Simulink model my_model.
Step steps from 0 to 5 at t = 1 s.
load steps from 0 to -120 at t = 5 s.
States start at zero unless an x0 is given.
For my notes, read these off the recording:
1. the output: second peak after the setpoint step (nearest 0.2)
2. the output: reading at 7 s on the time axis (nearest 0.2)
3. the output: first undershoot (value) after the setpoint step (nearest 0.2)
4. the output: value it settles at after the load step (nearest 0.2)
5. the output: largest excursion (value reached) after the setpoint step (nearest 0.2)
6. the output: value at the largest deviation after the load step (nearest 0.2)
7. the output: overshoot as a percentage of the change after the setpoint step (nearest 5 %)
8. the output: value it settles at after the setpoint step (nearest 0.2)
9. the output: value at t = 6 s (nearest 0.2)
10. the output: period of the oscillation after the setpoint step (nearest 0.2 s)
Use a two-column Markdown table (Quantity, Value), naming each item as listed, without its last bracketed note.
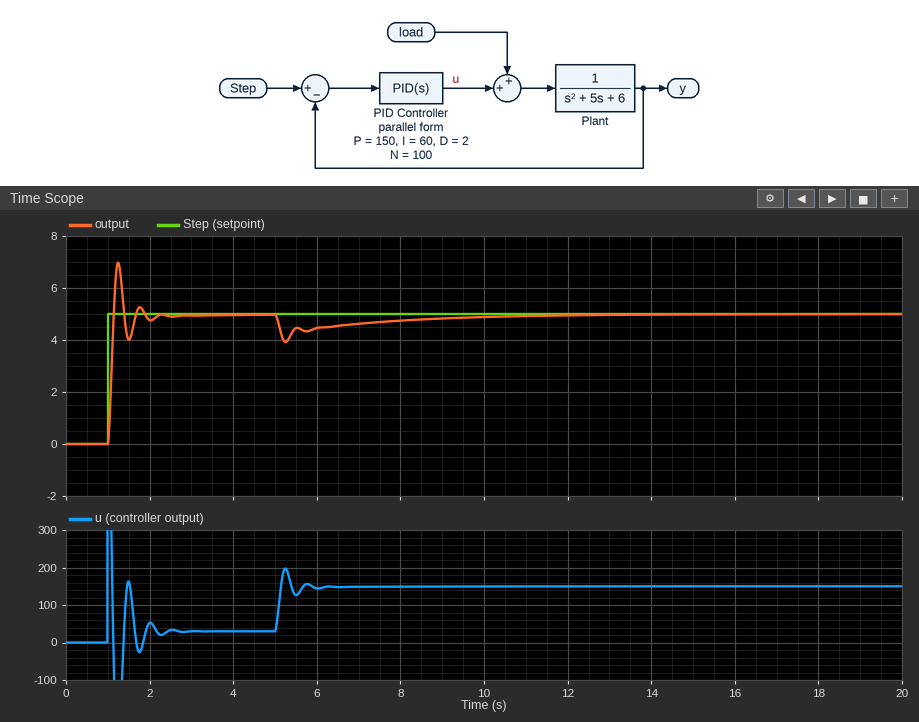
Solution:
| Quantity | Value |
|---|---|
| the output: second peak after the setpoint step | 5.2 |
| the output: reading at 7 s on the time axis | 4.6 |
| the output: first undershoot (value) after the setpoint step | 4.0 |
| the output: value it settles at after the load step | 5.0 |
| the output: largest excursion (value reached) after the setpoint step | 7.0 |
| the output: value at the largest deviation after the load step | 4.0 |
| the output: overshoot as a percentage of the change after the setpoint step | 40 % |
| the output: value it settles at after the setpoint step | 5.0 |
| the output: value at t = 6 s | 4.4 |
| the output: period of the oscillation after the setpoint step | 0.6 s |
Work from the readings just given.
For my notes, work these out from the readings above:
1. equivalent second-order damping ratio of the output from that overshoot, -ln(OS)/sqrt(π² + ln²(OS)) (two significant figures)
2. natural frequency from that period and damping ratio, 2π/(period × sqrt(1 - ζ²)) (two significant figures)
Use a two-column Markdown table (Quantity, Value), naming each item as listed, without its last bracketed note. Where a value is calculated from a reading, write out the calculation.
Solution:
| Quantity | Value |
|---|---|
| equivalent second-order damping ratio of the output from that overshoot, -ln(OS)/sqrt(π² + ln²(OS)) | ln(0.4) = -0.916; 0.916 / sqrt(9.870 + 0.840) = 0.28 |
| natural frequency from that period and damping ratio, 2π/(period × sqrt(1 - ζ²)) | 2π / (0.6 × sqrt(1 - 0.28²)) = 11 rad/s |
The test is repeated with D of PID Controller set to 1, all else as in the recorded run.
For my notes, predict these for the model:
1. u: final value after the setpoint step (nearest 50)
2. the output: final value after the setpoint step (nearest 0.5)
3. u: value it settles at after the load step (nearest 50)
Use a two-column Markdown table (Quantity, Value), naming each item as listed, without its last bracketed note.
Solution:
| Quantity | Value |
|---|---|
| u: final value after the setpoint step | 50 |
| the output: final value after the setpoint step | 5.0 |
| u: value it settles at after the load step | 150 |
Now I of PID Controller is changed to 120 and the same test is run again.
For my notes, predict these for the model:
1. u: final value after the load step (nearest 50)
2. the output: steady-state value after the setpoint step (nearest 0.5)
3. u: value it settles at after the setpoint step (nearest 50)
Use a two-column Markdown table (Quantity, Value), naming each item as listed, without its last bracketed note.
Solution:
| Quantity | Value |
|---|---|
| u: final value after the load step | 150 |
| the output: steady-state value after the setpoint step | 5.0 |
| u: value it settles at after the setpoint step | 50 |
